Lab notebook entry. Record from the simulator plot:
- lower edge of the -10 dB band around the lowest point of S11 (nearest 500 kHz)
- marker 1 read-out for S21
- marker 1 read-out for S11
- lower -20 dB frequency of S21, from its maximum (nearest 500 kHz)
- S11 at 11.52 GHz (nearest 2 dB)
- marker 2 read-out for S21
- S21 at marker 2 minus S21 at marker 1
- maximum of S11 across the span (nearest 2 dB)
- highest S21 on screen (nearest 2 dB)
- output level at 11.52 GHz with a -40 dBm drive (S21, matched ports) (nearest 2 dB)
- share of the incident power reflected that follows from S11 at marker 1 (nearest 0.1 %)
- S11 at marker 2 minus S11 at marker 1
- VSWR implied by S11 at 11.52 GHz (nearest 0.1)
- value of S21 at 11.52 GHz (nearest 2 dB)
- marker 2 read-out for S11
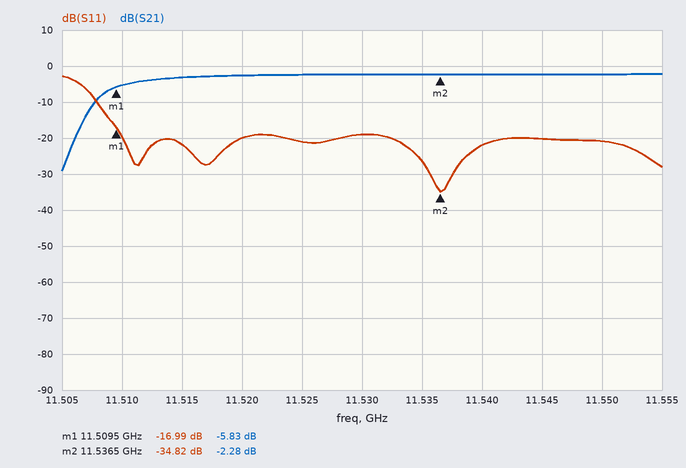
11.5080 GHz
-5.83 dB
-16.99 dB
11.5060 GHz
-20 dB
-2.28 dB
3.55 dB
-2 dB
-2 dB
-42 dBm
2.0 %
-17.83 dB
1.2
-2 dB
-34.82 dB
